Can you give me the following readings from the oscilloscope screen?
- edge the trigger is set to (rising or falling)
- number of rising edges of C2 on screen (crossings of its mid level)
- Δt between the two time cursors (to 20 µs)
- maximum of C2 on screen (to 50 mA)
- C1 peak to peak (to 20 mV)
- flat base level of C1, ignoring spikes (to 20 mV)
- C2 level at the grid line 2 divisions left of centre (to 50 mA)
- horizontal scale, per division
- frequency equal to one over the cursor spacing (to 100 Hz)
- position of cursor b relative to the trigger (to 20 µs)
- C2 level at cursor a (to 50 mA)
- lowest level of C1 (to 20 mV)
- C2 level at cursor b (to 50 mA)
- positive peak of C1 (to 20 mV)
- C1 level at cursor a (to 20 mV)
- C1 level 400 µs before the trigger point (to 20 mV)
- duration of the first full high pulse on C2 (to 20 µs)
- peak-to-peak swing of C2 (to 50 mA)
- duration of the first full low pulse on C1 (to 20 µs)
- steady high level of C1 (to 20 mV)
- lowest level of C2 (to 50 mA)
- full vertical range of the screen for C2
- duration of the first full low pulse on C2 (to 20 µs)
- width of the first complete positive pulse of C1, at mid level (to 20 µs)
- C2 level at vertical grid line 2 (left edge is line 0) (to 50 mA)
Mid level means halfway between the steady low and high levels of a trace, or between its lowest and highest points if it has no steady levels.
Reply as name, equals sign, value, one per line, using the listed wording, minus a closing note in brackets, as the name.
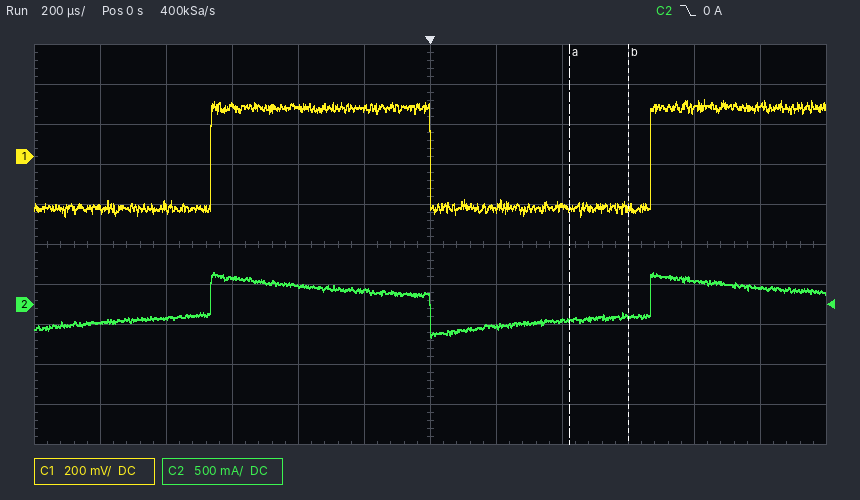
edge the trigger is set to = falling
number of rising edges of C2 on screen = 2
Δt between the two time cursors = 180 µs
maximum of C2 on screen = 400 mA
C1 peak to peak = 580 mV
flat base level of C1, ignoring spikes = -260 mV
C2 level at the grid line 2 divisions left of centre = 250 mA
horizontal scale, per division = 200 µs
frequency equal to one over the cursor spacing = 5.6 kHz
position of cursor b relative to the trigger = +600 µs
C2 level at cursor a = -200 mA
lowest level of C1 = -300 mV
C2 level at cursor b = -150 mA
positive peak of C1 = 280 mV
C1 level at cursor a = -260 mV
C1 level 400 µs before the trigger point = 240 mV
duration of the first full high pulse on C2 = 660 µs
peak-to-peak swing of C2 = 800 mA
duration of the first full low pulse on C1 = 660 µs
steady high level of C1 = 240 mV
lowest level of C2 = -400 mA
full vertical range of the screen for C2 = 5 A
duration of the first full low pulse on C2 = 660 µs
width of the first complete positive pulse of C1, at mid level = 660 µs
C2 level at vertical grid line 2 (left edge is line 0) = -150 mA
